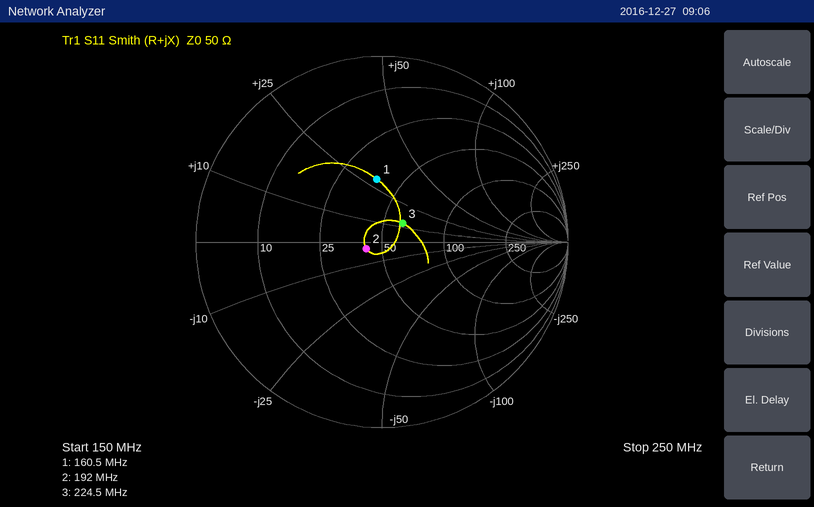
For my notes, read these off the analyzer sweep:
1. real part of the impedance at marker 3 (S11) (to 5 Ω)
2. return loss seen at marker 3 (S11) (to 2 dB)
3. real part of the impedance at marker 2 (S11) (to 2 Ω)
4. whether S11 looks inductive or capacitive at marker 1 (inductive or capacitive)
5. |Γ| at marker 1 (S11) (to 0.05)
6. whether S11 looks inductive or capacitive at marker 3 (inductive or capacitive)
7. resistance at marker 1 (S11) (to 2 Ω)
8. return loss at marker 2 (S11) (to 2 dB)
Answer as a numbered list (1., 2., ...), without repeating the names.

1. 60 Ω
2. 16 dB
3. 42 Ω
4. inductive
5. 0.35
6. inductive
7. 38 Ω
8. 20 dB
